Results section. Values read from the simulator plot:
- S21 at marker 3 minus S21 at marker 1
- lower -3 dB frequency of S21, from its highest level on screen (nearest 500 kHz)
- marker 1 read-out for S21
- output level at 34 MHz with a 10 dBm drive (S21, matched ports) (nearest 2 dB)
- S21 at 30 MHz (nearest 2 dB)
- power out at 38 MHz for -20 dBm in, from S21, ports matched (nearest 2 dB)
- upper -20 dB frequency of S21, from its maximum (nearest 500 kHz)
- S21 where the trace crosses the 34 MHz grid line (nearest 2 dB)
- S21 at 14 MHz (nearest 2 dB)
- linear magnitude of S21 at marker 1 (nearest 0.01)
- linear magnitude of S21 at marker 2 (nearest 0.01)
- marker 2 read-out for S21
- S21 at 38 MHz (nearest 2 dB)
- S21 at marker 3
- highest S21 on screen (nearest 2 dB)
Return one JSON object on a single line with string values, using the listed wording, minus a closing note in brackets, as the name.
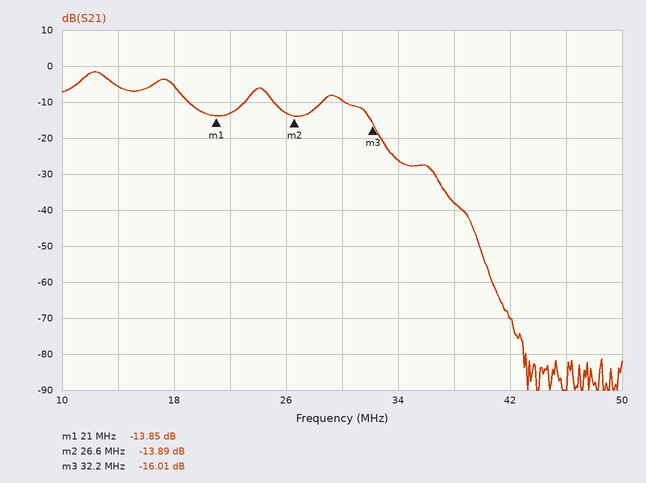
{"S21 at marker 3 minus S21 at marker 1": "-2.16 dB", "lower -3 dB frequency of S21, from its highest level on screen": "11.0 MHz", "marker 1 read-out for S21": "-13.85 dB", "output level at 34 MHz with a 10 dBm drive (S21, matched ports)": "-16 dBm", "S21 at 30 MHz": "-10 dB", "power out at 38 MHz for -20 dBm in, from S21, ports matched": "-58 dBm", "upper -20 dB frequency of S21, from its maximum": "33.0 MHz", "S21 where the trace crosses the 34 MHz grid line": "-26 dB", "S21 at 14 MHz": "-6 dB", "linear magnitude of S21 at marker 1": "0.20", "linear magnitude of S21 at marker 2": "0.20", "marker 2 read-out for S21": "-13.89 dB", "S21 at 38 MHz": "-38 dB", "S21 at marker 3": "-16.01 dB", "highest S21 on screen": "-2 dB"}
